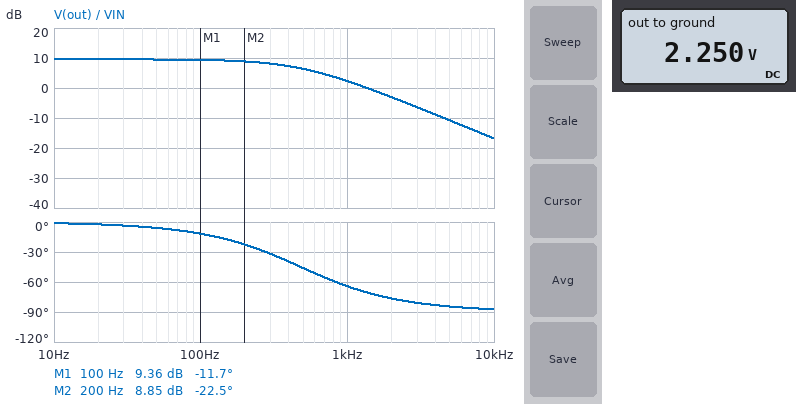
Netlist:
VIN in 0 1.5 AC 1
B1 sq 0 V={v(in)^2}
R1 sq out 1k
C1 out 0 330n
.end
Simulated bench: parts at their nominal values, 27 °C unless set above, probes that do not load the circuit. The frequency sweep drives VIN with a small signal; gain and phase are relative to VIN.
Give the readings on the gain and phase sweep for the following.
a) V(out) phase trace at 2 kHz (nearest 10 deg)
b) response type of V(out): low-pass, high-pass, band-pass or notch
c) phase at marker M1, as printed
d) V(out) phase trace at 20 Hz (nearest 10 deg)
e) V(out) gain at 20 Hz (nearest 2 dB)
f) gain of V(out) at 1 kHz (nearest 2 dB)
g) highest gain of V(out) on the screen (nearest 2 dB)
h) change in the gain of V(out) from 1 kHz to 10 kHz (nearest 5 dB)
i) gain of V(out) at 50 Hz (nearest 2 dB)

-80 deg
low-pass
-11.7 deg
0 deg
10 dB
2 dB
10 dB
-20 dB
10 dB
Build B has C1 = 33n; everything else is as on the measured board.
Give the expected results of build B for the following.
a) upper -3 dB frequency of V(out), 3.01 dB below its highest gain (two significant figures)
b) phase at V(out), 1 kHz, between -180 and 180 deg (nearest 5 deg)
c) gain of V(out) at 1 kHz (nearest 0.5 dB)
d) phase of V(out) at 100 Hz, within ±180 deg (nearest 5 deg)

4.8 kHz
-10 deg
9.5 dB
0 deg
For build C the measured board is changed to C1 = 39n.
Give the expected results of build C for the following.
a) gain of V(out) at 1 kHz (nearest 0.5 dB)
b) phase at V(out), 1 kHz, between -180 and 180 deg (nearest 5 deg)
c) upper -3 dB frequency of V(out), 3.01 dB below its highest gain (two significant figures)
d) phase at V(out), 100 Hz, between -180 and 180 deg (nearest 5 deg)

9.5 dB
-15 deg
4.1 kHz
0 deg
